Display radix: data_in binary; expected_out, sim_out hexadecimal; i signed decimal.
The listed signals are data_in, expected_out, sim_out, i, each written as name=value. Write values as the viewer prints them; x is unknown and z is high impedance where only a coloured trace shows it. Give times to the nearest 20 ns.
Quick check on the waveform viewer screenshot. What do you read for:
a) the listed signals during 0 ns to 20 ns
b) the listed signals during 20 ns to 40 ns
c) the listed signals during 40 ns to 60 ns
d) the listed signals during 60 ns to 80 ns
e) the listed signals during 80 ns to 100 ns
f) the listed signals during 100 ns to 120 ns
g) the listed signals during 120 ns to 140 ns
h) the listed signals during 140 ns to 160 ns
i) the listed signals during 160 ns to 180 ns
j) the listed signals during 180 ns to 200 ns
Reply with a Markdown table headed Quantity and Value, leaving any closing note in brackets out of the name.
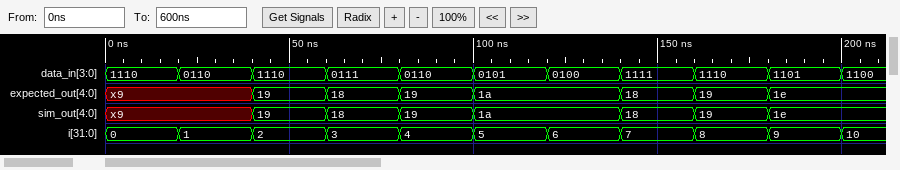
| Quantity | Value |
|---|---|
| the listed signals during 0 ns to 20 ns | data_in=1110, expected_out=x9, sim_out=x9, i=0 |
| the listed signals during 20 ns to 40 ns | data_in=0110, expected_out=x9, sim_out=x9, i=1 |
| the listed signals during 40 ns to 60 ns | data_in=1110, expected_out=19, sim_out=19, i=2 |
| the listed signals during 60 ns to 80 ns | data_in=0111, expected_out=18, sim_out=18, i=3 |
| the listed signals during 80 ns to 100 ns | data_in=0110, expected_out=19, sim_out=19, i=4 |
| the listed signals during 100 ns to 120 ns | data_in=0101, expected_out=1a, sim_out=1a, i=5 |
| the listed signals during 120 ns to 140 ns | data_in=0100, expected_out=1a, sim_out=1a, i=6 |
| the listed signals during 140 ns to 160 ns | data_in=1111, expected_out=18, sim_out=18, i=7 |
| the listed signals during 160 ns to 180 ns | data_in=1110, expected_out=19, sim_out=19, i=8 |
| the listed signals during 180 ns to 200 ns | data_in=1101, expected_out=1e, sim_out=1e, i=9 |
